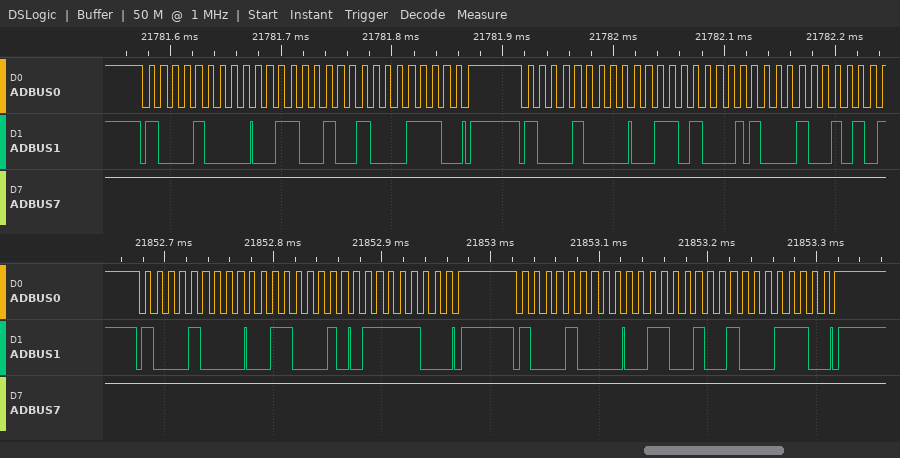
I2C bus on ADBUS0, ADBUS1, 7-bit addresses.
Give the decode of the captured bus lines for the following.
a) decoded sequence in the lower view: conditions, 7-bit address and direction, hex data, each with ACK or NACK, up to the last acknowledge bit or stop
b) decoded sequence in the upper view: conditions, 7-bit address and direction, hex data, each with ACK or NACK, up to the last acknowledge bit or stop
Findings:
start, address 44 write ACK, 31 ACK, 7C ACK, stop, start, address 44 write ACK, 32 ACK, 8E ACK, stop
start, address 44 write ACK, 32 ACK, 8E ACK, stop, start, address 44 write ACK, 34 ACK, repeated start, address 44 read ACK
